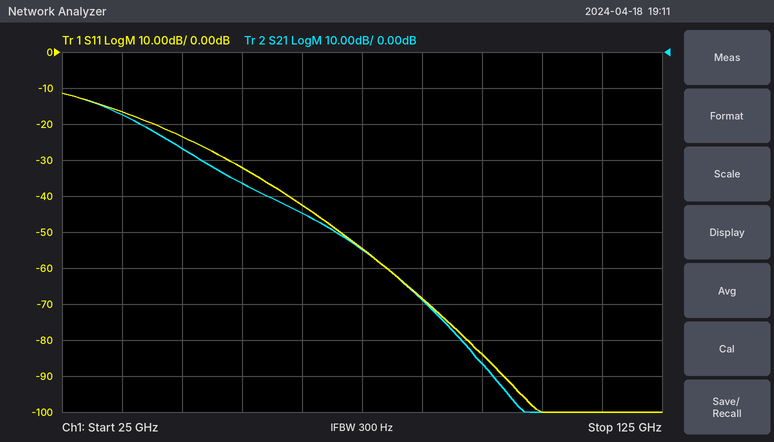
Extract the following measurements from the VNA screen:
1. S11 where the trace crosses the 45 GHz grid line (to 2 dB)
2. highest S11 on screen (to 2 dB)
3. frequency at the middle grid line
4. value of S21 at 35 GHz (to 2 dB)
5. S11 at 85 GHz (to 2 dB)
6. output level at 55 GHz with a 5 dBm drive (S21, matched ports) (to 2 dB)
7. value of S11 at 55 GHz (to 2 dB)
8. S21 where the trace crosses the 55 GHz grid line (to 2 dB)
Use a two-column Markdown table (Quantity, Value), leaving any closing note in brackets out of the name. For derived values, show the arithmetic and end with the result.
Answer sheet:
| Quantity | Value |
|---|---|
| S11 where the trace crosses the 45 GHz grid line | -24 dB |
| highest S11 on screen | -12 dB |
| frequency at the middle grid line | 75 GHz |
| value of S21 at 35 GHz | -18 dB |
| S11 at 85 GHz | -68 dB |
| output level at 55 GHz with a 5 dBm drive (S21, matched ports) | 5 dBm + (-36 dB) = -32 dBm |
| value of S11 at 55 GHz | -32 dB |
| S21 where the trace crosses the 55 GHz grid line | -36 dB |
